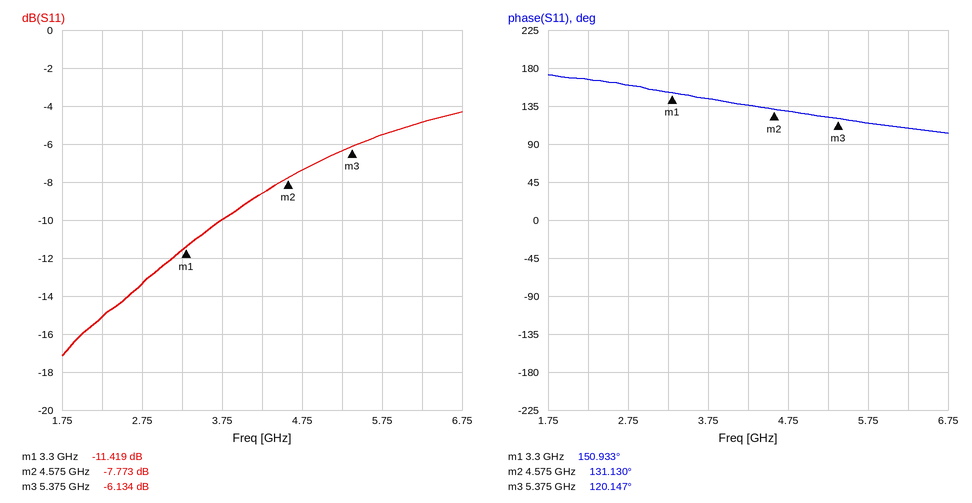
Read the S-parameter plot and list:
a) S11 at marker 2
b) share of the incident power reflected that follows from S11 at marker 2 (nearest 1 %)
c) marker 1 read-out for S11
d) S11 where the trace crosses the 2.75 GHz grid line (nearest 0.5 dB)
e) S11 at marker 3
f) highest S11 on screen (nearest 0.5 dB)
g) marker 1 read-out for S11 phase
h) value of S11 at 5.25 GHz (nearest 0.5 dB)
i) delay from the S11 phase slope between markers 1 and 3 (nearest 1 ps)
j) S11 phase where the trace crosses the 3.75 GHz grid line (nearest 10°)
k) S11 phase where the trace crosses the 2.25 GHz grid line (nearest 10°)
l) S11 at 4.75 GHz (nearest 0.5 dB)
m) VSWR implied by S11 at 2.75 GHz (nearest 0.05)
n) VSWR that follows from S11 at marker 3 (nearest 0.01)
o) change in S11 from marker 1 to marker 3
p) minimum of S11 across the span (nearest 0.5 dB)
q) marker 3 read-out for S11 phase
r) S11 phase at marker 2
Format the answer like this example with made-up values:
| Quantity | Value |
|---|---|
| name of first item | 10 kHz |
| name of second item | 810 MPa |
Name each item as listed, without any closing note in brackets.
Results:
| Quantity | Value |
|---|---|
| S11 at marker 2 | -7.773 dB |
| share of the incident power reflected that follows from S11 at marker 2 | 17 % |
| marker 1 read-out for S11 | -11.419 dB |
| S11 where the trace crosses the 2.75 GHz grid line | -13.5 dB |
| S11 at marker 3 | -6.134 dB |
| highest S11 on screen | -4.5 dB |
| marker 1 read-out for S11 phase | 150.933° |
| value of S11 at 5.25 GHz | -6.5 dB |
| delay from the S11 phase slope between markers 1 and 3 | 41 ps |
| S11 phase where the trace crosses the 3.75 GHz grid line | 140° |
| S11 phase where the trace crosses the 2.25 GHz grid line | 170° |
| S11 at 4.75 GHz | -7.5 dB |
| VSWR implied by S11 at 2.75 GHz | 1.55 |
| VSWR that follows from S11 at marker 3 | 2.95 |
| change in S11 from marker 1 to marker 3 | 5.285 dB |
| minimum of S11 across the span | -17.0 dB |
| marker 3 read-out for S11 phase | 120.147° |
| S11 phase at marker 2 | 131.130° |
